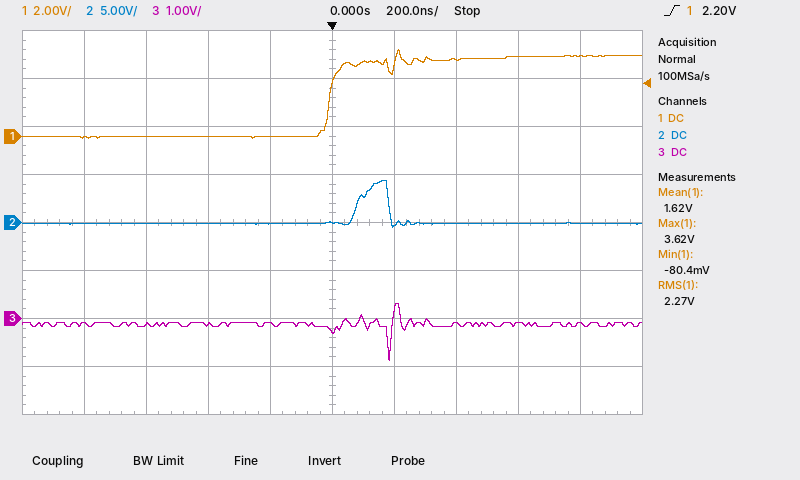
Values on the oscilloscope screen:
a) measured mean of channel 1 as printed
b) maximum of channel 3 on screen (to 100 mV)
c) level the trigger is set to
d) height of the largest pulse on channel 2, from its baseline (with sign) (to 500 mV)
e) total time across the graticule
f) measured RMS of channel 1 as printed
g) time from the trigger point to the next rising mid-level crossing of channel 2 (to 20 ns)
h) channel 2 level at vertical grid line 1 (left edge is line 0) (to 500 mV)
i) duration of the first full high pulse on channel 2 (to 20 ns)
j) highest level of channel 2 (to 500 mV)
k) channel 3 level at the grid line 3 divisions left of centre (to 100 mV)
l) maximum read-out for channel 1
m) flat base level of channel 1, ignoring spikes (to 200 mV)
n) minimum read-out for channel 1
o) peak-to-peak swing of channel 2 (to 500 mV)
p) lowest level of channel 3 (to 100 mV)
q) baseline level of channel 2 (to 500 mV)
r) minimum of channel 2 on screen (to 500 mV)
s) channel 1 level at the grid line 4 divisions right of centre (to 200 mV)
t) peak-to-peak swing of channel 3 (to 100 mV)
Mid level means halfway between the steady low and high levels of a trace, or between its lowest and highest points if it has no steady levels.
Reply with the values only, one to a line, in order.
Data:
1.62 V
300 mV
2.20 V
+4.5 V
2 µs
2.27 V
80 ns
0.0 V
100 ns
4.5 V
-100 mV
3.62 V
0.0 V
-80.4 mV
5.0 V
-900 mV
0.0 V
-500 mV
3.4 V
1.2 V
